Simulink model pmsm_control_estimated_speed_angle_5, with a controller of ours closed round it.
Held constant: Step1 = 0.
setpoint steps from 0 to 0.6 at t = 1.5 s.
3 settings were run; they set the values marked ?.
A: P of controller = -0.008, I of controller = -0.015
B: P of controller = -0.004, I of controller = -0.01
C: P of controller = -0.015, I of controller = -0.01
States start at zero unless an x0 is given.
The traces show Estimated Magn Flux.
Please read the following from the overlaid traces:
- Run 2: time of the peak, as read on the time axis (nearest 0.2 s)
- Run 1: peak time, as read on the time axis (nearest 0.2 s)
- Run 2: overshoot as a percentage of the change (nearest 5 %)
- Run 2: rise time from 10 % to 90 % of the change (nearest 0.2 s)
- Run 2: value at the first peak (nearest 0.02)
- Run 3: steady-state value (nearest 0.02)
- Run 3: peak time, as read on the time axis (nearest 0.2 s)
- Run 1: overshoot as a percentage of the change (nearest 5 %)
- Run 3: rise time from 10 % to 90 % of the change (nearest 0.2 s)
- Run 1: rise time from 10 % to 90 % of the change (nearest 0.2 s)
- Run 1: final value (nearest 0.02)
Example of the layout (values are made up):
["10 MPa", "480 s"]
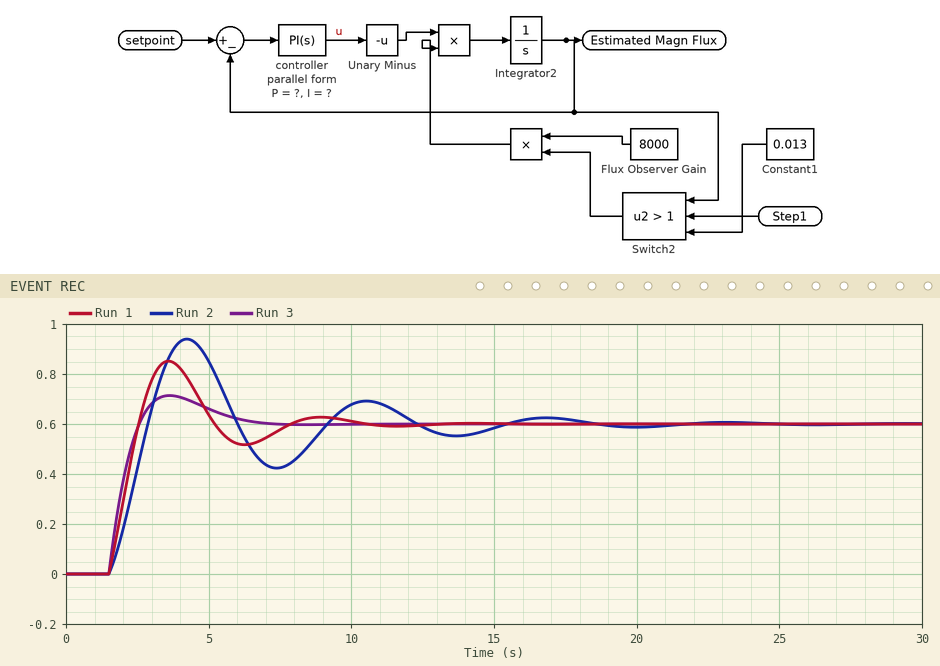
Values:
["4.2 s", "3.6 s", "55 %", "1.0 s", "0.94", "0.60", "3.6 s", "40 %", "0.8 s", "0.8 s", "0.60"]
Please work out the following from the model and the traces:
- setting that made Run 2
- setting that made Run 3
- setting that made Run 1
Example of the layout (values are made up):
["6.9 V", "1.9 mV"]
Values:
["B", "C", "A"]
